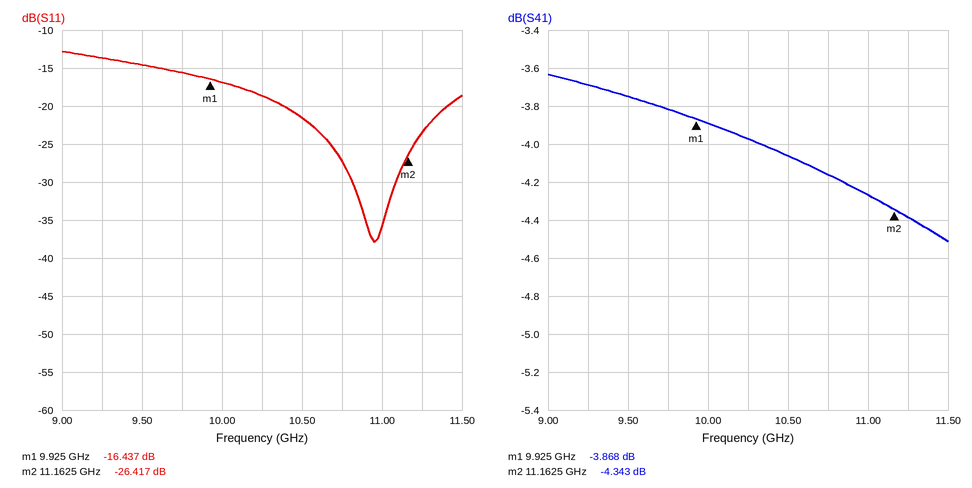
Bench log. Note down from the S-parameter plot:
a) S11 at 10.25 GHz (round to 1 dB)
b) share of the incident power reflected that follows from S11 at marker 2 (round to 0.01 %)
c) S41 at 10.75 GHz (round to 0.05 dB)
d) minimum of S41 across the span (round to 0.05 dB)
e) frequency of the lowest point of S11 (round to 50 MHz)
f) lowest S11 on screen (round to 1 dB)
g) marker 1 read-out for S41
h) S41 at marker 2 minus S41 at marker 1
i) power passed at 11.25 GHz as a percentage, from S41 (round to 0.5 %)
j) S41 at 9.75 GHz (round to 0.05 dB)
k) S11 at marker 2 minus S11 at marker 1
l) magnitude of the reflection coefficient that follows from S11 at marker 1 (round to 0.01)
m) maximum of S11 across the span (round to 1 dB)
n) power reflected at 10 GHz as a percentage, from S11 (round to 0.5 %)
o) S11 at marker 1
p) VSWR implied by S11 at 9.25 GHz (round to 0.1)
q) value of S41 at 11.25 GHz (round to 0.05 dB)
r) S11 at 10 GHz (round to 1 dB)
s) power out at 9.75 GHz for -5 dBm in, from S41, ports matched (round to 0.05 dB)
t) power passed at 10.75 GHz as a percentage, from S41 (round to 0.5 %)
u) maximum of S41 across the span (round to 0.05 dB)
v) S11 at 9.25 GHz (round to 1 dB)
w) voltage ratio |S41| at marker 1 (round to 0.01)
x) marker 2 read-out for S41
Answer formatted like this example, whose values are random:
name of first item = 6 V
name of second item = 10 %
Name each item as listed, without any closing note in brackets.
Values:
S11 at 10.25 GHz = -19 dB
share of the incident power reflected that follows from S11 at marker 2 = 0.23 %
S41 at 10.75 GHz = -4.15 dB
minimum of S41 across the span = -4.50 dB
frequency of the lowest point of S11 = 10.95 GHz
lowest S11 on screen = -38 dB
marker 1 read-out for S41 = -3.868 dB
S41 at marker 2 minus S41 at marker 1 = -0.475 dB
power passed at 11.25 GHz as a percentage, from S41 = 36.5 %
S41 at 9.75 GHz = -3.80 dB
S11 at marker 2 minus S11 at marker 1 = -9.980 dB
magnitude of the reflection coefficient that follows from S11 at marker 1 = 0.15
maximum of S11 across the span = -13 dB
power reflected at 10 GHz as a percentage, from S11 = 2.0 %
S11 at marker 1 = -16.437 dB
VSWR implied by S11 at 9.25 GHz = 1.5
value of S41 at 11.25 GHz = -4.40 dB
S11 at 10 GHz = -17 dB
power out at 9.75 GHz for -5 dBm in, from S41, ports matched = -8.80 dBm
power passed at 10.75 GHz as a percentage, from S41 = 38.5 %
maximum of S41 across the span = -3.65 dB
S11 at 9.25 GHz = -14 dB
voltage ratio |S41| at marker 1 = 0.64
marker 2 read-out for S41 = -4.343 dB
